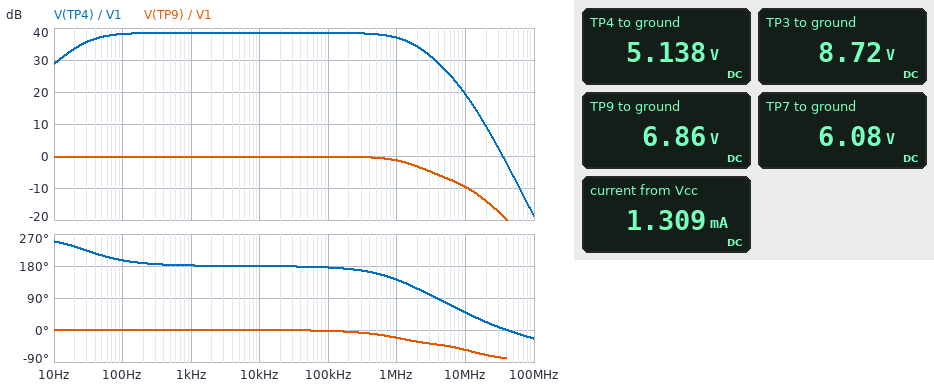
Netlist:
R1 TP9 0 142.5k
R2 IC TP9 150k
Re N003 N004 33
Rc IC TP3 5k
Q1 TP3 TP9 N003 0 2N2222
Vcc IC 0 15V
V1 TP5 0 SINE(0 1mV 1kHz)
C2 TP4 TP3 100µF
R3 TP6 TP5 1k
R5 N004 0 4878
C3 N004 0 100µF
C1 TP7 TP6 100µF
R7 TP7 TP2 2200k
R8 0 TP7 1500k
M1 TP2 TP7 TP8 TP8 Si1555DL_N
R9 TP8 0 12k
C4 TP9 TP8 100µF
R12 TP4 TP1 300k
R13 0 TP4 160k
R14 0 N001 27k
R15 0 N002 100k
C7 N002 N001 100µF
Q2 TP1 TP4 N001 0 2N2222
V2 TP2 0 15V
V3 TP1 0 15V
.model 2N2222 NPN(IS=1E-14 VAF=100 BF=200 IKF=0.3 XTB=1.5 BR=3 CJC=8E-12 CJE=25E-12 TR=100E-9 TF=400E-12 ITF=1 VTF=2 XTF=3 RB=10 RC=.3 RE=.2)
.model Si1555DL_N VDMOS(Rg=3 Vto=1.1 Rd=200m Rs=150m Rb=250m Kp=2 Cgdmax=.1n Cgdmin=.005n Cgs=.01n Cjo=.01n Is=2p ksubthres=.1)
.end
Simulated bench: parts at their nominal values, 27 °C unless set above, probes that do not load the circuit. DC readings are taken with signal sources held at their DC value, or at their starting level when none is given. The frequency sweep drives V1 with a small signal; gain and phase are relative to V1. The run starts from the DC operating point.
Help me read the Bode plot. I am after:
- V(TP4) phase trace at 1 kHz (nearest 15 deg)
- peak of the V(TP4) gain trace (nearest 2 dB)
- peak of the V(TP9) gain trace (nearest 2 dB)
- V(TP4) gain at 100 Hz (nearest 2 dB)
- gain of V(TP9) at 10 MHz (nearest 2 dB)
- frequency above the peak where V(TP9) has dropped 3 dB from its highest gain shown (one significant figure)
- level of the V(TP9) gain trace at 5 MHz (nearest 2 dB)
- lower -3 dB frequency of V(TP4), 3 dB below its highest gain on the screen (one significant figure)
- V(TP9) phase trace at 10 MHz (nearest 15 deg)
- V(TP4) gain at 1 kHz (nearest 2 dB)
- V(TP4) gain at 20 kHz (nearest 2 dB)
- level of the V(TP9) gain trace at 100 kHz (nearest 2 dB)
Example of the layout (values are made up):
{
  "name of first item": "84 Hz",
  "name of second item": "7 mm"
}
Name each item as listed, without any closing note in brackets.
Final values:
{
  "V(TP4) phase trace at 1 kHz": "180 deg",
  "peak of the V(TP4) gain trace": "38 dB",
  "peak of the V(TP9) gain trace": "0 dB",
  "V(TP4) gain at 100 Hz": "38 dB",
  "gain of V(TP9) at 10 MHz": "-10 dB",
  "frequency above the peak where V(TP9) has dropped 3 dB from its highest gain shown": "2 MHz",
  "level of the V(TP9) gain trace at 5 MHz": "-6 dB",
  "lower -3 dB frequency of V(TP4), 3 dB below its highest gain on the screen": "30 Hz",
  "V(TP9) phase trace at 10 MHz": "-60 deg",
  "V(TP4) gain at 1 kHz": "38 dB",
  "V(TP4) gain at 20 kHz": "38 dB",
  "level of the V(TP9) gain trace at 100 kHz": "0 dB"
}
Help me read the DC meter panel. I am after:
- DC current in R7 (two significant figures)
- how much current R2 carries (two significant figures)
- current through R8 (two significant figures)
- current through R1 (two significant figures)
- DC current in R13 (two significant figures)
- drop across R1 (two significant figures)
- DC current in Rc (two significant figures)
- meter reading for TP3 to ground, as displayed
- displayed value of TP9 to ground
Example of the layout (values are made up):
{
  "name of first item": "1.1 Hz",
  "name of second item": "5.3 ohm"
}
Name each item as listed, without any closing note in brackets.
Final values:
{
  "DC current in R7": "4.1 µA",
  "how much current R2 carries": "54 µA",
  "current through R8": "4.1 µA",
  "current through R1": "48 µA",
  "DC current in R13": "32 µA",
  "drop across R1": "6.9 V",
  "DC current in Rc": "1.3 mA",
  "meter reading for TP3 to ground, as displayed": "8.72 V",
  "displayed value of TP9 to ground": "6.86 V"
}
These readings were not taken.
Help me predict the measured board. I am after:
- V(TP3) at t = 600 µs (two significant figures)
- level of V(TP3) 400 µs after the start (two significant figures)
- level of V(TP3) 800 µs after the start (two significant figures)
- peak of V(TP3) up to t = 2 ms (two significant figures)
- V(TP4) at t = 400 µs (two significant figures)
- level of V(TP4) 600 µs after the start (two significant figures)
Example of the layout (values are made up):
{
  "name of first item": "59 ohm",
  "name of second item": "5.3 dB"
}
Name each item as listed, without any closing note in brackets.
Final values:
{
  "V(TP3) at t = 600 µs": "8.8 V",
  "level of V(TP3) 400 µs after the start": "8.7 V",
  "level of V(TP3) 800 µs after the start": "8.8 V",
  "peak of V(TP3) up to t = 2 ms": "8.8 V",
  "V(TP4) at t = 400 µs": "5.1 V",
  "level of V(TP4) 600 µs after the start": "5.2 V"
}
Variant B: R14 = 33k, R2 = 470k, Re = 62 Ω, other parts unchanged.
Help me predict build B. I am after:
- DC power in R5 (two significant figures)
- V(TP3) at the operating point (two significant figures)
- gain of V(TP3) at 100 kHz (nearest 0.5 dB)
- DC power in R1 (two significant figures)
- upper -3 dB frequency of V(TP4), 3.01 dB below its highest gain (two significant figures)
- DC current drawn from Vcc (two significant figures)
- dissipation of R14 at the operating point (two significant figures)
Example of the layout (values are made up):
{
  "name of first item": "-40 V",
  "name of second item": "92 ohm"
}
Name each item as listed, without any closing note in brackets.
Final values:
{
  "DC power in R5": "1.3 mW",
  "V(TP3) at the operating point": "12 V",
  "gain of V(TP3) at 100 kHz": "32.5 dB",
  "DC power in R1": "73 µW",
  "upper -3 dB frequency of V(TP4), 3.01 dB below its highest gain": "2.9 MHz",
  "DC current drawn from Vcc": "550 µA",
  "dissipation of R14 at the operating point": "630 µW"
}
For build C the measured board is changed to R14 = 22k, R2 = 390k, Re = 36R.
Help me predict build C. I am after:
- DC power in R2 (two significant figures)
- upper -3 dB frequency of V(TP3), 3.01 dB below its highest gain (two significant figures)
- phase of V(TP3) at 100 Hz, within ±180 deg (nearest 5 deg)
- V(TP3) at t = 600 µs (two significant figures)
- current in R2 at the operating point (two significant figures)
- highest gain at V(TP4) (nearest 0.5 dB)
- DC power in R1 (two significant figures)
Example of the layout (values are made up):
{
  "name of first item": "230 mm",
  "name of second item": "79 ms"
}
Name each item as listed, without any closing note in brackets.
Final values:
{
  "DC power in R2": "330 µW",
  "upper -3 dB frequency of V(TP3), 3.01 dB below its highest gain": "2.5 MHz",
  "phase of V(TP3) at 100 Hz, within ±180 deg": "-170 deg",
  "V(TP3) at t = 600 µs": "12 V",
  "current in R2 at the operating point": "29 µA",
  "highest gain at V(TP4)": "35.5 dB",
  "DC power in R1": "97 µW"
}
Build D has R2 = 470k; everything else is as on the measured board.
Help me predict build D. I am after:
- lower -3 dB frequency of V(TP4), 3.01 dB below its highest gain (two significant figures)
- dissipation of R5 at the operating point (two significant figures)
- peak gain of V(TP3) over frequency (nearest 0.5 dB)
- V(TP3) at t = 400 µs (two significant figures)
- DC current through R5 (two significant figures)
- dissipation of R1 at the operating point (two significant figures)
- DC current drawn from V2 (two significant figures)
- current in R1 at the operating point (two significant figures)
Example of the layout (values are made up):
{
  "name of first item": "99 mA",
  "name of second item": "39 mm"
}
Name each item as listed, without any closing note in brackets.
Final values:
{
  "lower -3 dB frequency of V(TP4), 3.01 dB below its highest gain": "19 Hz",
  "dissipation of R5 at the operating point": "1.4 mW",
  "peak gain of V(TP3) over frequency": "35.0 dB",
  "V(TP3) at t = 400 µs": "12 V",
  "DC current through R5": "530 µA",
  "dissipation of R1 at the operating point": "73 µW",
  "DC current drawn from V2": "430 µA",
  "current in R1 at the operating point": "23 µA"
}
